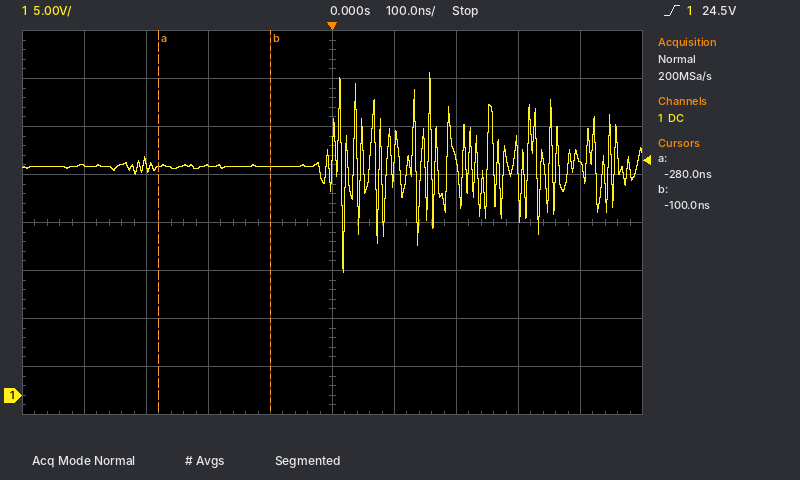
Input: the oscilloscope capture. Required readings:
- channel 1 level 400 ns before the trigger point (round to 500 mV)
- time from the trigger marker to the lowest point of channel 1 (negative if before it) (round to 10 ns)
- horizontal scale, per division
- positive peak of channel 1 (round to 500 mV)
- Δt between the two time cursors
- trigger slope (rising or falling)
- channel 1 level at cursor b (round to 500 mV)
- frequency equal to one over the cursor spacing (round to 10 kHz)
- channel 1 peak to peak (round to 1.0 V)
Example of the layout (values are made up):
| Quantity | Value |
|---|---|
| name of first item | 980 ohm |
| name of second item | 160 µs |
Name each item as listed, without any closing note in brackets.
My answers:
| Quantity | Value |
|---|---|
| channel 1 level 400 ns before the trigger point | 24.0 V |
| time from the trigger marker to the lowest point of channel 1 (negative if before it) | +20 ns |
| horizontal scale, per division | 100 ns |
| positive peak of channel 1 | 33.5 V |
| Δt between the two time cursors | 180 ns |
| trigger slope | rising |
| channel 1 level at cursor b | 24.0 V |
| frequency equal to one over the cursor spacing | 5.56 MHz |
| channel 1 peak to peak | 21.0 V |
